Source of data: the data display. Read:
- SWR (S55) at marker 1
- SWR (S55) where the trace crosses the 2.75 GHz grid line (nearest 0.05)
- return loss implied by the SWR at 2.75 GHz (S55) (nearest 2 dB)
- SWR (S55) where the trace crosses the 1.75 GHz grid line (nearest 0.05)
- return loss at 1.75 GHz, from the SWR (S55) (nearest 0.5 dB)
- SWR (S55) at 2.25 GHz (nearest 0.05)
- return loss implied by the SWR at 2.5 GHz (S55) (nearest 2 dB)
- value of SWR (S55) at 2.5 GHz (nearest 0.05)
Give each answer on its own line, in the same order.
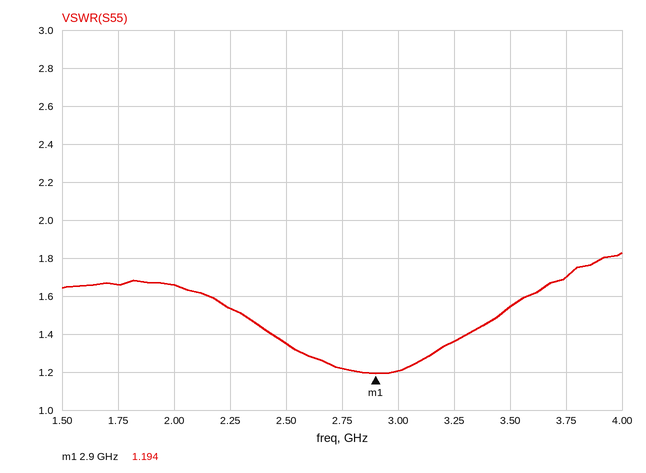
1.194
1.20
20 dB
1.65
12.0 dB
1.55
16 dB
1.35
